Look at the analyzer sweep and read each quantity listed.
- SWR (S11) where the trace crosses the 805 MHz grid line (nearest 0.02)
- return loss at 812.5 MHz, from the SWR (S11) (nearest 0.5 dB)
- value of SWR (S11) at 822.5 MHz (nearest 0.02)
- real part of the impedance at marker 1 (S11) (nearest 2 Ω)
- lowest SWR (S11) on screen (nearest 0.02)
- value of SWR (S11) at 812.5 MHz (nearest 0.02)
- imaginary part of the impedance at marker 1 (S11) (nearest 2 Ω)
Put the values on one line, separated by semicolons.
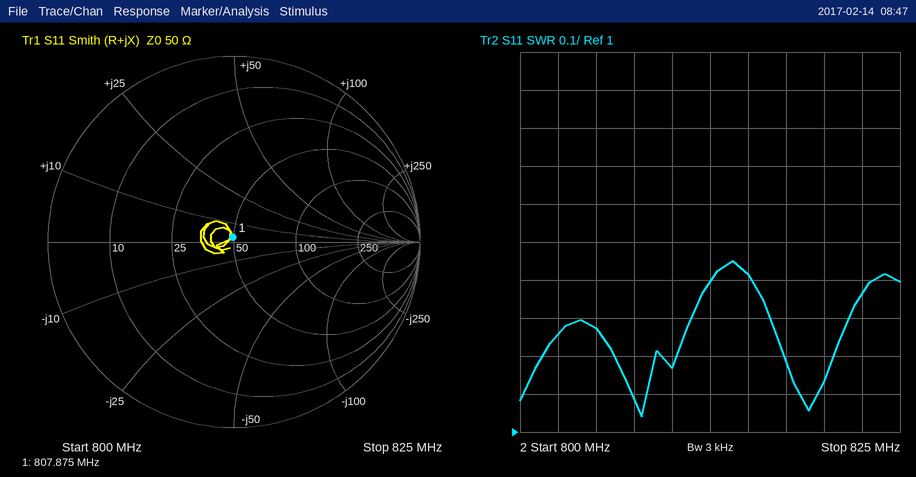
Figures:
1.28; 15.5 dB; 1.36; 50 Ω; 1.04; 1.40; +2 Ω
